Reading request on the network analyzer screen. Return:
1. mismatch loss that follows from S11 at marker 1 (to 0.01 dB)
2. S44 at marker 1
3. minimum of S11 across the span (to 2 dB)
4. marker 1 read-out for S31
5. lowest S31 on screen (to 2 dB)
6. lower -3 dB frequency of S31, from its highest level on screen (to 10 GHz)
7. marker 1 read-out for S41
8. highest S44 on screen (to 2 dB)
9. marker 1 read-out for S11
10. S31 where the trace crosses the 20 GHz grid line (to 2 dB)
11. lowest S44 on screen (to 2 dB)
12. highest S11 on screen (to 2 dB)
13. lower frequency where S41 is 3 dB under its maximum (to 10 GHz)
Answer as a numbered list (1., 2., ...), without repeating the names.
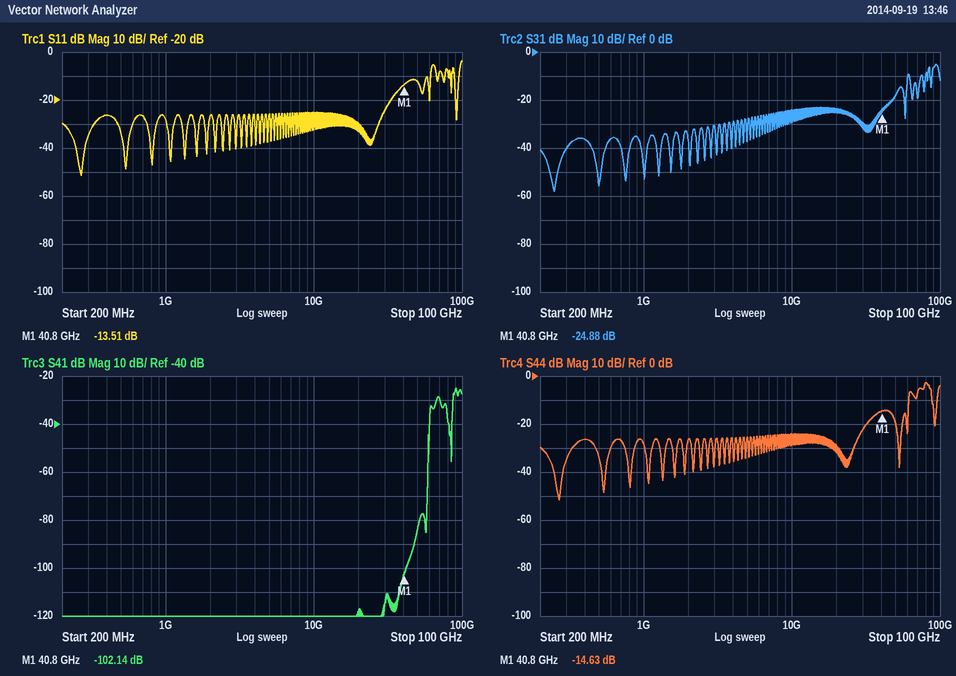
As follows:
1. 0.20 dB
2. -14.63 dB
3. -52 dB
4. -24.88 dB
5. -58 dB
6. 90 GHz
7. -102.14 dB
8. -2 dB
9. -13.51 dB
10. -24 dB
11. -52 dB
12. -4 dB
13. 90 GHz
